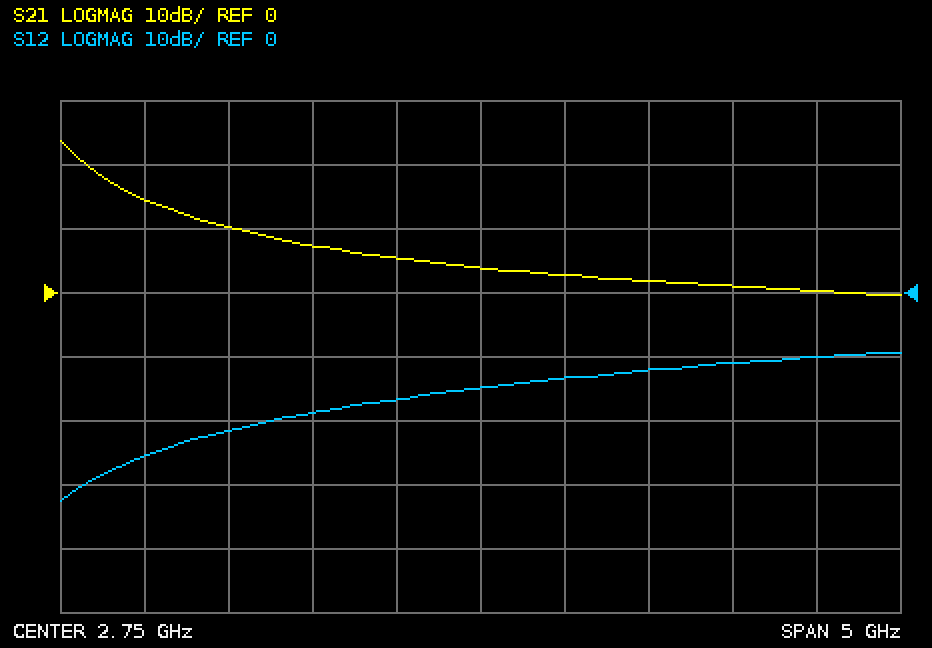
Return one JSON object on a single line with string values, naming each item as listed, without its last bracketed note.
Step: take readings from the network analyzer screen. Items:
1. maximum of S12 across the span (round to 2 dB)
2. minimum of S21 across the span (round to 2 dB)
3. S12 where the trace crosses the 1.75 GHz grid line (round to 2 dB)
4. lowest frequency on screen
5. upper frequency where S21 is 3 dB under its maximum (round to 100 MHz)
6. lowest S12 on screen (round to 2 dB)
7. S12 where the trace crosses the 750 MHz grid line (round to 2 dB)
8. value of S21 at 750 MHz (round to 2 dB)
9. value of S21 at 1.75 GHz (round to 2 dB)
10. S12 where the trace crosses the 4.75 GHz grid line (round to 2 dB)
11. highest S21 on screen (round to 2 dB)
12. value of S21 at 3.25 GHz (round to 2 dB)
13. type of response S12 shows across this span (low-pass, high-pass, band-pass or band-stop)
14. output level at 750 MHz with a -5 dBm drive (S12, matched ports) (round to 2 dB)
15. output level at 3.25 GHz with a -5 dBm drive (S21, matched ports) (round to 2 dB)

{"maximum of S12 across the span": "-10 dB", "minimum of S21 across the span": "0 dB", "S12 where the trace crosses the 1.75 GHz grid line": "-18 dB", "lowest frequency on screen": "250 MHz", "upper frequency where S21 is 3 dB under its maximum": "400 MHz", "lowest S12 on screen": "-32 dB", "S12 where the trace crosses the 750 MHz grid line": "-26 dB", "value of S21 at 750 MHz": "14 dB", "value of S21 at 1.75 GHz": "8 dB", "S12 where the trace crosses the 4.75 GHz grid line": "-10 dB", "highest S21 on screen": "24 dB", "value of S21 at 3.25 GHz": "2 dB", "type of response S12 shows across this span": "high-pass", "output level at 750 MHz with a -5 dBm drive (S12, matched ports)": "-30 dBm", "output level at 3.25 GHz with a -5 dBm drive (S21, matched ports)": "-2 dBm"}
